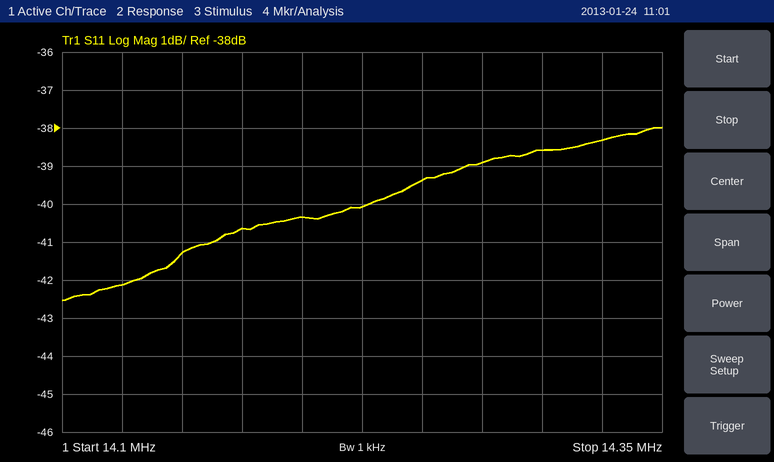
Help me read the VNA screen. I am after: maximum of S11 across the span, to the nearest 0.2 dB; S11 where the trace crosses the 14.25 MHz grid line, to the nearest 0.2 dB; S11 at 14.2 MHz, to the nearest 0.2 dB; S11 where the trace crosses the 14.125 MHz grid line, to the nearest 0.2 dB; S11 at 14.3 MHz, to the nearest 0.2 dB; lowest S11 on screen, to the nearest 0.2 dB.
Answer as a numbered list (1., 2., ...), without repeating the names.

1. -38.0 dB
2. -39.4 dB
3. -40.4 dB
4. -42.2 dB
5. -38.6 dB
6. -42.6 dB
